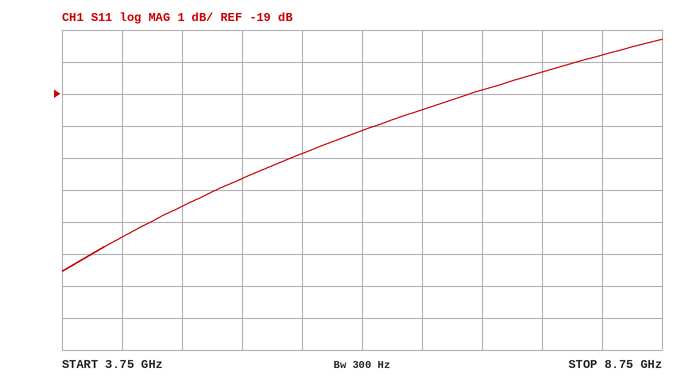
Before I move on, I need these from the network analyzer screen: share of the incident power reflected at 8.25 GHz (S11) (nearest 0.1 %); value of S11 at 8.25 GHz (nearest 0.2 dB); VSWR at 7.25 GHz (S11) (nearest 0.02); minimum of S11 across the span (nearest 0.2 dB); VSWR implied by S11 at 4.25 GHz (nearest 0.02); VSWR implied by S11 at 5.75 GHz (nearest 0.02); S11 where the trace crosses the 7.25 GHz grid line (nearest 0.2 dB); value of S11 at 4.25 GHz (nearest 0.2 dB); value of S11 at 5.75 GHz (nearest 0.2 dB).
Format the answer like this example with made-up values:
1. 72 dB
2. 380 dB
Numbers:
1. 1.7 %
2. -17.8 dB
3. 1.26
4. -24.6 dB
5. 1.14
6. 1.20
7. -18.8 dB
8. -23.4 dB
9. -20.8 dB
